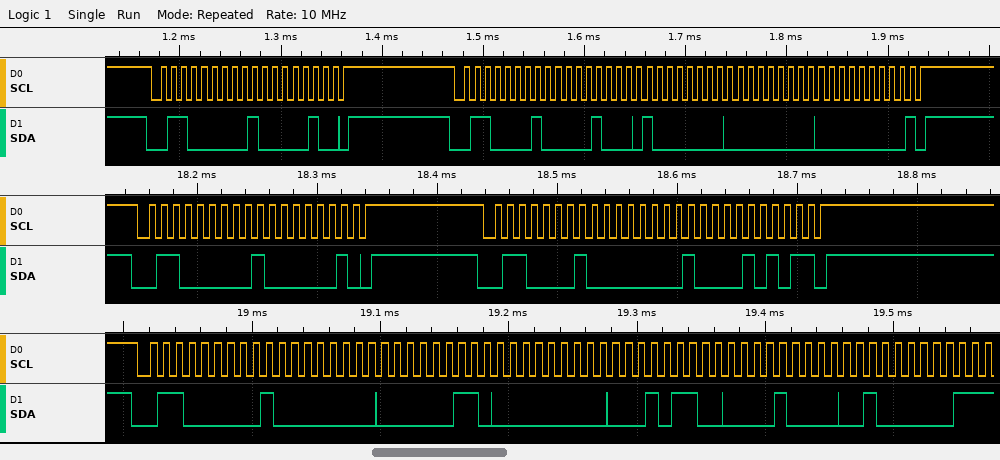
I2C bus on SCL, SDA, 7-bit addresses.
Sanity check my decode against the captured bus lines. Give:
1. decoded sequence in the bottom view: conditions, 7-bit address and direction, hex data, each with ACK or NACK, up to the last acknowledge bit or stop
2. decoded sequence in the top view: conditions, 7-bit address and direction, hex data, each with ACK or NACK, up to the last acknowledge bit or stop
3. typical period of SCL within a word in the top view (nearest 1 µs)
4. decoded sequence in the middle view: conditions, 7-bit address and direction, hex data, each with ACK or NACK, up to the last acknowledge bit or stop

start, address 30 write ACK, 80 ACK, 03 ACK, 00 ACK, 16 ACK, 08 ACK, 20 ACK
start, address 30 write ACK, 82 ACK, stop, start, address 30 read ACK, 08 ACK, 80 ACK, 00 ACK, 00 NACK, stop
10 µs
start, address 30 write ACK, 81 ACK, stop, start, address 30 read ACK, 01 ACK, 15 NACK, stop
